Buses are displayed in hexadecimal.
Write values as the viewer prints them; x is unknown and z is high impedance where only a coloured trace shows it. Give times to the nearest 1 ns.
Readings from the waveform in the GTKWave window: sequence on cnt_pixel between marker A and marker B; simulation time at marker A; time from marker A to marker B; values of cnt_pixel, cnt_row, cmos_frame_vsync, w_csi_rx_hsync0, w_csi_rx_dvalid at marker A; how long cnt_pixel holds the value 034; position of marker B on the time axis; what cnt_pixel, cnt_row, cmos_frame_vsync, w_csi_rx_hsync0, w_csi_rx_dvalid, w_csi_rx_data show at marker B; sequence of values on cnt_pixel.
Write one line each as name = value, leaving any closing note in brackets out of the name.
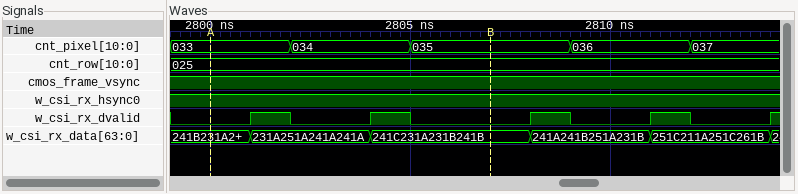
sequence on cnt_pixel between marker A and marker B = 033, 034, 035
simulation time at marker A = 2800 ns
time from marker A to marker B = 7 ns
values of cnt_pixel, cnt_row, cmos_frame_vsync, w_csi_rx_hsync0, w_csi_rx_dvalid at marker A = cnt_pixel=033, cnt_row=025, cmos_frame_vsync=1, w_csi_rx_hsync0=1, w_csi_rx_dvalid=0
how long cnt_pixel holds the value 034 = 3 ns
position of marker B on the time axis = 2807 ns
what cnt_pixel, cnt_row, cmos_frame_vsync, w_csi_rx_hsync0, w_csi_rx_dvalid, w_csi_rx_data show at marker B = cnt_pixel=035, cnt_row=025, cmos_frame_vsync=1, w_csi_rx_hsync0=1, w_csi_rx_dvalid=0, w_csi_rx_data=241C231A231B241B
sequence of values on cnt_pixel = 033, 034, 035, 036, 037
